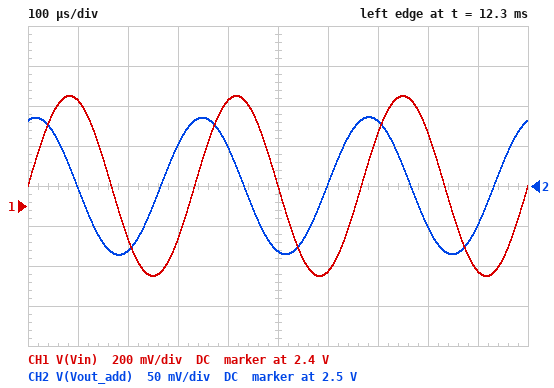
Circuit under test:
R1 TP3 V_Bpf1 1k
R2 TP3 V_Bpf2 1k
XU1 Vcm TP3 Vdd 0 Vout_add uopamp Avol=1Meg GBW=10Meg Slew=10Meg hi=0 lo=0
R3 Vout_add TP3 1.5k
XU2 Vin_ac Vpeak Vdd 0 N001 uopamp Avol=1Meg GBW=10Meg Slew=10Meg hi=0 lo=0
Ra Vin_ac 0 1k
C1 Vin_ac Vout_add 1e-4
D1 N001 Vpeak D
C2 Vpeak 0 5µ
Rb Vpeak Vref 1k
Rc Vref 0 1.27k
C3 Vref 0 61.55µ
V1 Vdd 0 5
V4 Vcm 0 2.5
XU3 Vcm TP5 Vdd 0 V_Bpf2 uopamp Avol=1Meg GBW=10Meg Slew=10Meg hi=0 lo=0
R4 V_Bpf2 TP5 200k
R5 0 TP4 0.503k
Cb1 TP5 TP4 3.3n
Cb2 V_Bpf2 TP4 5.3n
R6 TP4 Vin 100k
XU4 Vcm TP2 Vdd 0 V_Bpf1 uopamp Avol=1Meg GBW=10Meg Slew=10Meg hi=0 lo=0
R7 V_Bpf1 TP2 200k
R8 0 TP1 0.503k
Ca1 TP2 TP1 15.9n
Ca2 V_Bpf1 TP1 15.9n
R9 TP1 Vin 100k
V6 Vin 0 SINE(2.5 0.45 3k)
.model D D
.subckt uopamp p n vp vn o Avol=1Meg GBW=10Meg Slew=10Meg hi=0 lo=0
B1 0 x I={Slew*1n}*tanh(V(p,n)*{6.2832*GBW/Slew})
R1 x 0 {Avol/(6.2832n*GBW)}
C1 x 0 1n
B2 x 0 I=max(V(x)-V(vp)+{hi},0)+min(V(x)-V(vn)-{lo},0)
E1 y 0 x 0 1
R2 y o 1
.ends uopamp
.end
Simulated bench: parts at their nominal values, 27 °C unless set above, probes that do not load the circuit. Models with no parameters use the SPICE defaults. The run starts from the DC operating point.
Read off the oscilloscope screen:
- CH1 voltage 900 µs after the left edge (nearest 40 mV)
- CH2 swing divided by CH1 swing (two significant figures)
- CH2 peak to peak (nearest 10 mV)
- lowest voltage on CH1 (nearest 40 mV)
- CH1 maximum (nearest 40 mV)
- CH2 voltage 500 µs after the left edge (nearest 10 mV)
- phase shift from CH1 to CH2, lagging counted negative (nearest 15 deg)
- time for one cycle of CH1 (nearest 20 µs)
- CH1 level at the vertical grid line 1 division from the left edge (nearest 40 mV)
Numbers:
2.08 V
0.19
170 mV
2.04 V
2.96 V
2.42 V
75 deg
340 µs
2.92 V
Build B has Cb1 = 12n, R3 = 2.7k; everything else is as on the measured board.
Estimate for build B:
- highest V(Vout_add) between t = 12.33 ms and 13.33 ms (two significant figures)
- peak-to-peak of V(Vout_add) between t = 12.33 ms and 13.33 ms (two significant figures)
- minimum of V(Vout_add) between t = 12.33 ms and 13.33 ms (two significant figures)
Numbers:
2.8 V
520 mV
2.2 V
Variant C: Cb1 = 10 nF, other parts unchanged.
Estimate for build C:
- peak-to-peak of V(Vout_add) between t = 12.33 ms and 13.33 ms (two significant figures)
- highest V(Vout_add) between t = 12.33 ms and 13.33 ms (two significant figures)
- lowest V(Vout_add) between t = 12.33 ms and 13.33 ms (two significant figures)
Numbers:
330 mV
2.7 V
2.3 V
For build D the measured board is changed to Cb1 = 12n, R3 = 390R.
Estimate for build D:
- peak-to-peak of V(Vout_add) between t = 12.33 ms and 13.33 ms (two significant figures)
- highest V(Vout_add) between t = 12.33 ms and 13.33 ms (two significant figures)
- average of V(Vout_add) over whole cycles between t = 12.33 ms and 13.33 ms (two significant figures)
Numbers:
75 mV
2.5 V
2.5 V
